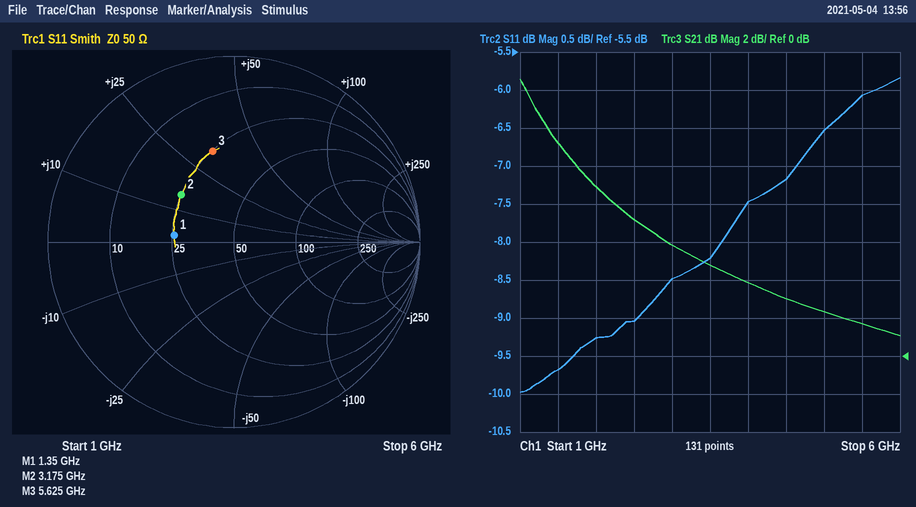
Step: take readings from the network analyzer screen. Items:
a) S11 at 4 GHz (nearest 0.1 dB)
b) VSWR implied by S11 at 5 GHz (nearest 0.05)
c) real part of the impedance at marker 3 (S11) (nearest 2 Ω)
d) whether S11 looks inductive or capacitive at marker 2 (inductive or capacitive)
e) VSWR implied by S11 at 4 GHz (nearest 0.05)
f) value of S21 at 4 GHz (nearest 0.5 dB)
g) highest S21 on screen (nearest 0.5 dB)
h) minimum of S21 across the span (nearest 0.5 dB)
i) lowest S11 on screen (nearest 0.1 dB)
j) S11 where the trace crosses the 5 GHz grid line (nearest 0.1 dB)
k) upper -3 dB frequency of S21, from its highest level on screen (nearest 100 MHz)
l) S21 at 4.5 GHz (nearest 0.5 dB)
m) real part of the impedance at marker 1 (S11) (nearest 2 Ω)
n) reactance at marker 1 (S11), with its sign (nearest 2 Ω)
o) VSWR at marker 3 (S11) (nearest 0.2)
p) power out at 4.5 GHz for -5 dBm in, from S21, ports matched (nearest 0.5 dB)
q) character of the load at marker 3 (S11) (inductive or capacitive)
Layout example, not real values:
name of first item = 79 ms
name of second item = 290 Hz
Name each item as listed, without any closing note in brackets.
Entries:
S11 at 4 GHz = -7.5 dB
VSWR implied by S11 at 5 GHz = 2.80
real part of the impedance at marker 3 (S11) = 26 Ω
whether S11 looks inductive or capacitive at marker 2 = inductive
VSWR implied by S11 at 4 GHz = 2.45
value of S21 at 4 GHz = 4.0 dB
highest S21 on screen = 14.5 dB
minimum of S21 across the span = 1.0 dB
lowest S11 on screen = -10.0 dB
S11 where the trace crosses the 5 GHz grid line = -6.5 dB
upper -3 dB frequency of S21, from its highest level on screen = 1.4 GHz
S21 at 4.5 GHz = 3.0 dB
real part of the impedance at marker 1 (S11) = 26 Ω
reactance at marker 1 (S11), with its sign = +2 Ω
VSWR at marker 3 (S11) = 3.0
power out at 4.5 GHz for -5 dBm in, from S21, ports matched = -2.0 dBm
character of the load at marker 3 (S11) = inductive
